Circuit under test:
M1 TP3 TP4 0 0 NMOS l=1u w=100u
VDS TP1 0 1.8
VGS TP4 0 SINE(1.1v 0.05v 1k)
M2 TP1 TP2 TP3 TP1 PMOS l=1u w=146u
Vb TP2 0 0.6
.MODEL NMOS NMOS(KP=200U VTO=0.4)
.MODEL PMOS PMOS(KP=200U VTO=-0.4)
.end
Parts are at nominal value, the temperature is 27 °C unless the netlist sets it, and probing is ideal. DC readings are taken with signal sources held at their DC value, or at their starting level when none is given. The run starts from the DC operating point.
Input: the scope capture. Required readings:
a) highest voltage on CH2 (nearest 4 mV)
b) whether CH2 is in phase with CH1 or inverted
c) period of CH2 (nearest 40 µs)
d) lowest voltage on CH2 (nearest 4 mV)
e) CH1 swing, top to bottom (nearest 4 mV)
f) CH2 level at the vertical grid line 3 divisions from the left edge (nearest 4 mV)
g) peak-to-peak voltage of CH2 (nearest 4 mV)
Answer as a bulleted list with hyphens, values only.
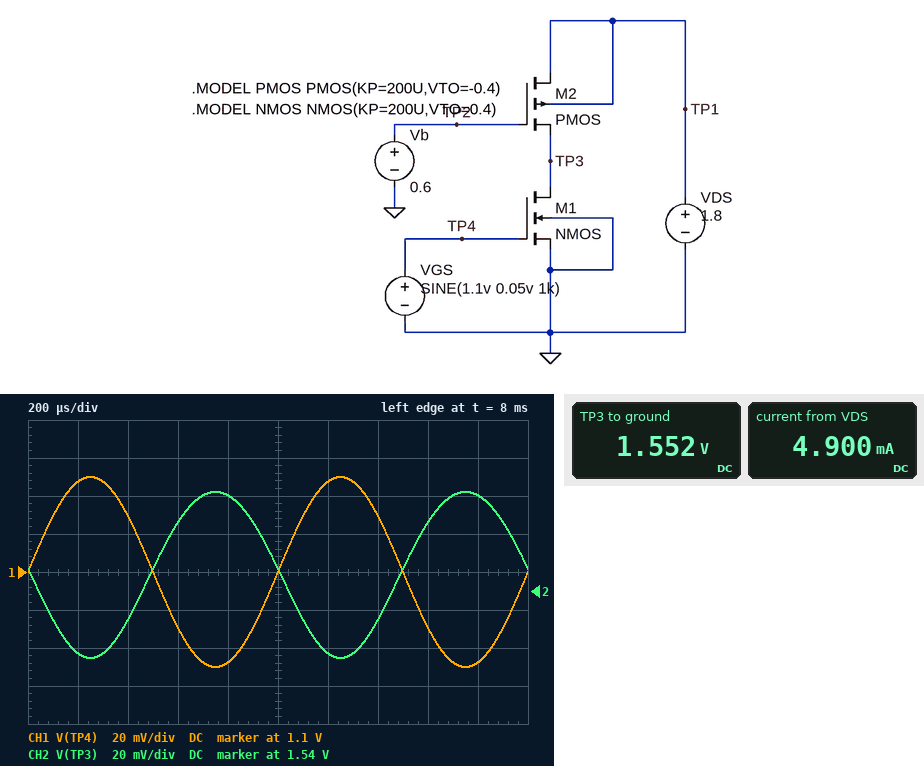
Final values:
- 1.592 V
- inverted
- 1.00 ms
- 1.504 V
- 100 mV
- 1.576 V
- 88 mV
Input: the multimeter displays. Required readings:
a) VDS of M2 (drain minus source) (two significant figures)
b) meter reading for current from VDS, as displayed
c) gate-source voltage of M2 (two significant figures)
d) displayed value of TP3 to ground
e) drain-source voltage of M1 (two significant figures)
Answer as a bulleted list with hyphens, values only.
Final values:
- 250 mV
- 4.900 mA
- -950 mV
- 1.552 V
- 1.6 V
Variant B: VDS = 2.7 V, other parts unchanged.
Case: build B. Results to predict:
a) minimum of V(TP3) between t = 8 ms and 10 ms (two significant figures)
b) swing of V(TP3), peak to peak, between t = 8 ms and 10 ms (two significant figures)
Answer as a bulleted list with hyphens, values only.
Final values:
- 2.6 V
- 30 mV
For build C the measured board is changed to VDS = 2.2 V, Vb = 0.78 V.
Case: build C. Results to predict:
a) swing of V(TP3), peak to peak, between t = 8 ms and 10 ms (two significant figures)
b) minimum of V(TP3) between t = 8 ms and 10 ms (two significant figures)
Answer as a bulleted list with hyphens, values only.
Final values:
- 57 mV
- 2.0 V
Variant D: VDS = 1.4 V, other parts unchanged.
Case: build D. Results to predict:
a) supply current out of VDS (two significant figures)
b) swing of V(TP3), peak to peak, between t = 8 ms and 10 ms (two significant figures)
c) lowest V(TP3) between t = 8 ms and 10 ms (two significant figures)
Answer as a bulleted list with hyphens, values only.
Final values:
- 2.3 mA
- 39 mV
- 180 mV
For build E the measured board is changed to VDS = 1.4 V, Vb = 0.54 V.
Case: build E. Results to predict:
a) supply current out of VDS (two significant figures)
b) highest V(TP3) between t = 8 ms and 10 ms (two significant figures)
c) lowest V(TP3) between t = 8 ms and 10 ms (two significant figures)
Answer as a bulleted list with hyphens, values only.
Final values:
- 3.1 mA
- 310 mV
- 250 mV
